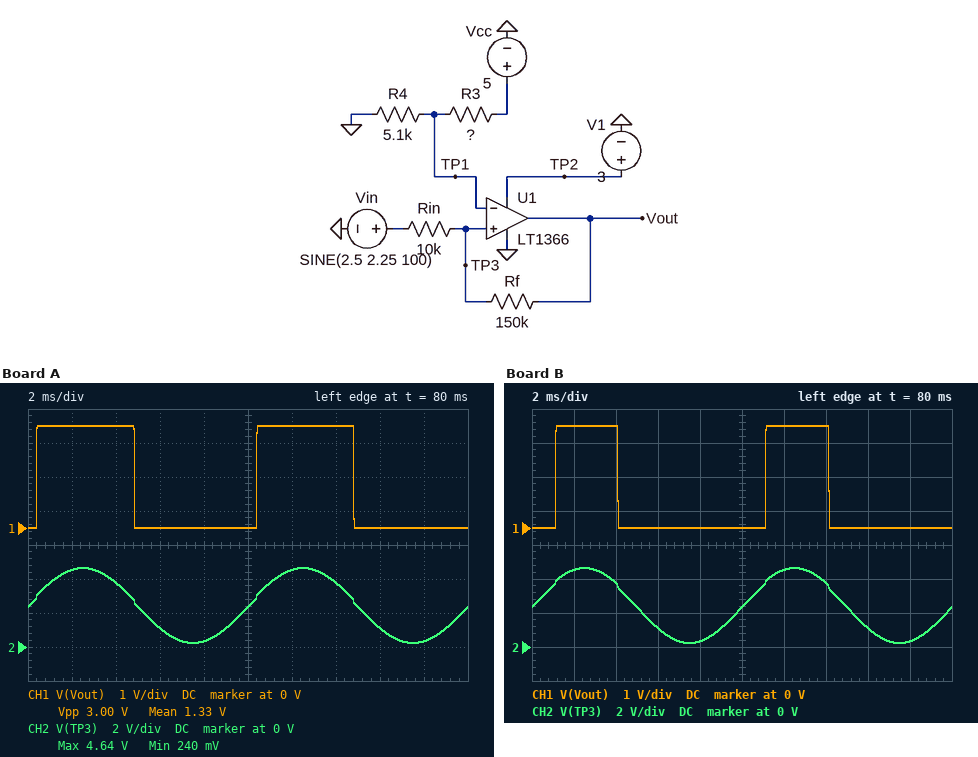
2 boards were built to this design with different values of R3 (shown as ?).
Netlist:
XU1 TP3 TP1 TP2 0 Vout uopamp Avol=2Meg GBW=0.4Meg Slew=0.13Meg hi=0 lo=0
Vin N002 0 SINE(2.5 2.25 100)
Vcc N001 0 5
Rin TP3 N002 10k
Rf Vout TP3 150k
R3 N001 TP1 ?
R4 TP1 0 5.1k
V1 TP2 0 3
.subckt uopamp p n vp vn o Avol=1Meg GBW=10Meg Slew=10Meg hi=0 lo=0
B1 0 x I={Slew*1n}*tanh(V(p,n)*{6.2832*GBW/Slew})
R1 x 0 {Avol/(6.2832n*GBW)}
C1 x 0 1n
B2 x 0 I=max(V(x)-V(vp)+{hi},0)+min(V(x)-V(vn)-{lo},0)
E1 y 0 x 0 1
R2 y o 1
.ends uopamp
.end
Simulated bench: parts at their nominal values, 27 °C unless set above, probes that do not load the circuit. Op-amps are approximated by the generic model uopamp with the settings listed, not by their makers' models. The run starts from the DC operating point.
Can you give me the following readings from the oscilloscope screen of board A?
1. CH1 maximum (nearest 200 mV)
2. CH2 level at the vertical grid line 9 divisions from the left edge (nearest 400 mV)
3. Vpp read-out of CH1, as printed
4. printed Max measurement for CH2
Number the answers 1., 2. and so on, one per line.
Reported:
1. 3.0 V
2. 400 mV
3. 3.00 V
4. 4.64 V
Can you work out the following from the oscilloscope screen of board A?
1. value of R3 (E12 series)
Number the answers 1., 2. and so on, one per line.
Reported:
1. 3.9 kΩ
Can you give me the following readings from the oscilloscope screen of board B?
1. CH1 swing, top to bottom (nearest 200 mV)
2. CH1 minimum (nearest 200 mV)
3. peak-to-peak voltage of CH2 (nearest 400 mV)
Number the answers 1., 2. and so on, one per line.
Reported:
1. 3.0 V
2. 0 V
3. 4.4 V
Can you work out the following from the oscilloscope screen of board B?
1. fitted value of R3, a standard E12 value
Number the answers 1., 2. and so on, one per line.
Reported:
1. 1.8 kΩ
